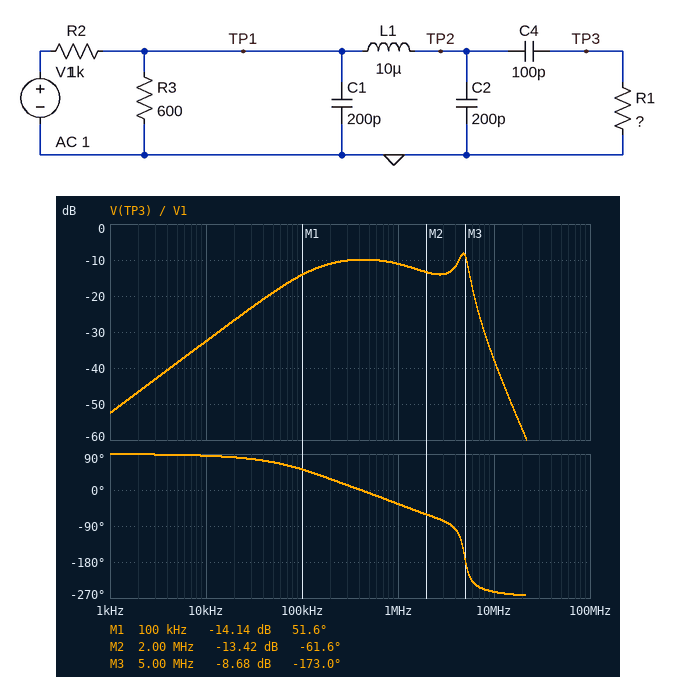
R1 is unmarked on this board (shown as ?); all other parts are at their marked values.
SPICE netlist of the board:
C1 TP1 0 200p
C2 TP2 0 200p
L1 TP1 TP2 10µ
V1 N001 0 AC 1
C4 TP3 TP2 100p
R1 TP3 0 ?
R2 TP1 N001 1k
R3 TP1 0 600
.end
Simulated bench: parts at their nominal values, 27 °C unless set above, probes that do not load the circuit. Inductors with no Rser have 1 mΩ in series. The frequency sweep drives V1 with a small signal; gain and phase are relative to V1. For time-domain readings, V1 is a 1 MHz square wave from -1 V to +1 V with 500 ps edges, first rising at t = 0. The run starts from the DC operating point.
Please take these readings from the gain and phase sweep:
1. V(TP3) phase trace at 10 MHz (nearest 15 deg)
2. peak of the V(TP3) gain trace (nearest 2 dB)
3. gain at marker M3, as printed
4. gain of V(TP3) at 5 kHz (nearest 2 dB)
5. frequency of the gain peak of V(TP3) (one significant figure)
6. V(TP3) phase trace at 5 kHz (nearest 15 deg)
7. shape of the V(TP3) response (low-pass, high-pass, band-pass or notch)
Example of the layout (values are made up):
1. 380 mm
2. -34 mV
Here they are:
1. -255 deg
2. -8 dB
3. -8.68 dB
4. -38 dB
5. 5 MHz
6. 90 deg
7. band-pass
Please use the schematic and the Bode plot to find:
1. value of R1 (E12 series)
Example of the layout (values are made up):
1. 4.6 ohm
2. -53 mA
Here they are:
1. 10 kΩ
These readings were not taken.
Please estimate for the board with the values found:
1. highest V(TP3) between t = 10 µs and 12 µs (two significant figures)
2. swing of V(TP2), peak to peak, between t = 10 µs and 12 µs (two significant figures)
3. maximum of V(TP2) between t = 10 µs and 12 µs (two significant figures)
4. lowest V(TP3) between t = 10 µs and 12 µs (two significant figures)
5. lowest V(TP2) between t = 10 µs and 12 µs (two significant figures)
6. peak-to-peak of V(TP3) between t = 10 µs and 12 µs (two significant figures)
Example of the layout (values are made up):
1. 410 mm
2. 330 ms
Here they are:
1. 370 mV
2. 740 mV
3. 370 mV
4. -370 mV
5. -370 mV
6. 740 mV
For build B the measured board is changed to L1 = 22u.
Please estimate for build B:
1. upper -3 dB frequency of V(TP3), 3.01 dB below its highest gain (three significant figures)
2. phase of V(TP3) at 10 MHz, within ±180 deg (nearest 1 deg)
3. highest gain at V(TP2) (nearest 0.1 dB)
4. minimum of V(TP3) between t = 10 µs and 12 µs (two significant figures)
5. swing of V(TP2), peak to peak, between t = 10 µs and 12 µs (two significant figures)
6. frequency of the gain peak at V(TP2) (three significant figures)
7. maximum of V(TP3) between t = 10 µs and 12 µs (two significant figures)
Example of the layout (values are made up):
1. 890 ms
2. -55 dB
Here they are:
1. 3.53 MHz
2. 104 deg
3. -7.3 dB
4. -430 mV
5. 810 mV
6. 3.08 MHz
7. 430 mV
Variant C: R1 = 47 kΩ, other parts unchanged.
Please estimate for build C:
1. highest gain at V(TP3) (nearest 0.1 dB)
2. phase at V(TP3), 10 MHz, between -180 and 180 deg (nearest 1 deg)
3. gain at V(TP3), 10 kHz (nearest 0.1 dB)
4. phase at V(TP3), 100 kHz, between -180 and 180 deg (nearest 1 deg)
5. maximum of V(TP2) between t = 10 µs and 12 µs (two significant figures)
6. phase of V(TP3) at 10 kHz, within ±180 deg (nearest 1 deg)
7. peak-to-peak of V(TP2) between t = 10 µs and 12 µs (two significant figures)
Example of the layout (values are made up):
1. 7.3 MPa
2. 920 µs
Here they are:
1. -7.8 dB
2. 104 deg
3. -19.5 dB
4. 13 deg
5. 380 mV
6. 73 deg
7. 760 mV
